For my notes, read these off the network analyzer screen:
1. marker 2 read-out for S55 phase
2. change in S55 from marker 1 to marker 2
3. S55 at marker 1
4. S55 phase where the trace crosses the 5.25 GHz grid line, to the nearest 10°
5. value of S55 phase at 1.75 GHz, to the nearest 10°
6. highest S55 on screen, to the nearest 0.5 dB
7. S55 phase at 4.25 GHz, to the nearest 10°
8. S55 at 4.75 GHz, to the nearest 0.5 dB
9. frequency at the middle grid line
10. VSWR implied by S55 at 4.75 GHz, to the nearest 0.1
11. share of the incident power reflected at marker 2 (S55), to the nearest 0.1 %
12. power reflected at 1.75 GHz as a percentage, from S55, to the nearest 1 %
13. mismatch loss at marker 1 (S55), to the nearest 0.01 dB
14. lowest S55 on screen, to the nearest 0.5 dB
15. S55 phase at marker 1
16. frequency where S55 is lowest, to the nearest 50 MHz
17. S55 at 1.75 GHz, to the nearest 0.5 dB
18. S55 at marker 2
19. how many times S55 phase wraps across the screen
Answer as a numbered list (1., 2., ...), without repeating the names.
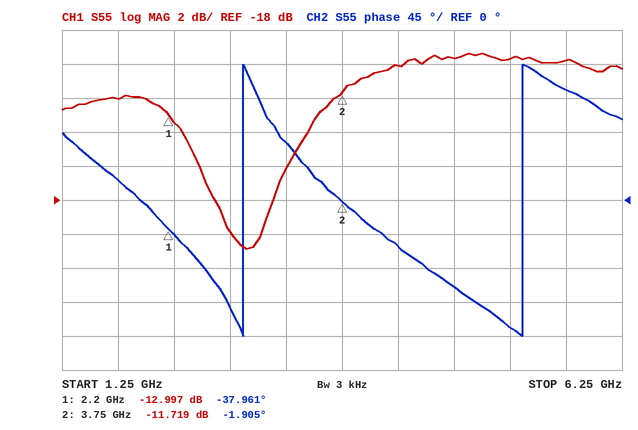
1. -1.905°
2. 1.278 dB
3. -12.997 dB
4. -170°
5. 30°
6. -9.5 dB
7. -60°
8. -9.5 dB
9. 3.75 GHz
10. 2.0
11. 6.7 %
12. 6 %
13. 0.22 dB
14. -21.0 dB
15. -37.961°
16. 2.90 GHz
17. -12.0 dB
18. -11.719 dB
19. 2
